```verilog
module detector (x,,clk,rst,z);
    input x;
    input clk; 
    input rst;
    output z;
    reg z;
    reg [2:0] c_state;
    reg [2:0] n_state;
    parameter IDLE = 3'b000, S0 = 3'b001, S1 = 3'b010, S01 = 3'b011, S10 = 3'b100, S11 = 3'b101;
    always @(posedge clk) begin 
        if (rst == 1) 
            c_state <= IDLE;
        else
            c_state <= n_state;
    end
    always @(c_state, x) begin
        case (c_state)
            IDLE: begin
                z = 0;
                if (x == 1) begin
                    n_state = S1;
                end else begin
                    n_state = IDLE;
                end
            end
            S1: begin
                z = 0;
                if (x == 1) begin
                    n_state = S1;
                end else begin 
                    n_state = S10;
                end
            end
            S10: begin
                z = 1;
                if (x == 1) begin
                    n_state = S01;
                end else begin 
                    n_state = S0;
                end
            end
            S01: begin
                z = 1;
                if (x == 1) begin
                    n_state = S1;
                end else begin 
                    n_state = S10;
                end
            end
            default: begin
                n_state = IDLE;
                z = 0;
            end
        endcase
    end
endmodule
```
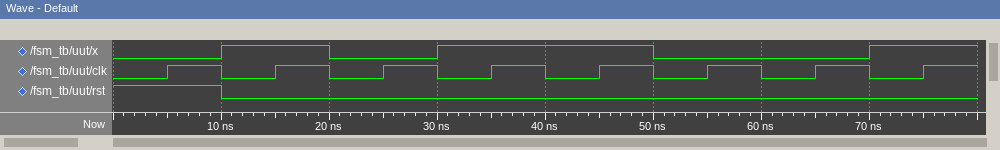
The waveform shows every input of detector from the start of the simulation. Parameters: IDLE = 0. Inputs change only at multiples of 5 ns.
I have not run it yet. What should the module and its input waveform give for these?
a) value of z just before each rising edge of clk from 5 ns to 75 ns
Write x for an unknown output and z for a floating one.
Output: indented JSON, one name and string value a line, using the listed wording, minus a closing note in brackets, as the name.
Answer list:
{
  "value of z just before each rising edge of clk from 5 ns to 75 ns": "0 0 0 1 1 0 1 0"
}
